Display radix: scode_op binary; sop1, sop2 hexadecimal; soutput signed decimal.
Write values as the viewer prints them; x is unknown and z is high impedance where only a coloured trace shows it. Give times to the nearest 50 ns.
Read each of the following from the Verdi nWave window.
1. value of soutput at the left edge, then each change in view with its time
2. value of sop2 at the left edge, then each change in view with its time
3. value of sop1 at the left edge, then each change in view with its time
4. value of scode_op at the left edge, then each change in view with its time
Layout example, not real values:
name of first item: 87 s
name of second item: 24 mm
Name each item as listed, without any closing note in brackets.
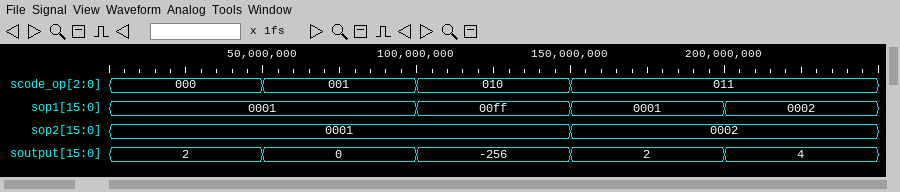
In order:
value of soutput at the left edge, then each change in view with its time: 2, 0 at 50 ns, -256 at 100 ns, 2 at 150 ns, 4 at 200 ns
value of sop2 at the left edge, then each change in view with its time: 0001, 0002 at 150 ns
value of sop1 at the left edge, then each change in view with its time: 0001, 00ff at 100 ns, 0001 at 150 ns, 0002 at 200 ns
value of scode_op at the left edge, then each change in view with its time: 000, 001 at 50 ns, 010 at 100 ns, 011 at 150 ns
